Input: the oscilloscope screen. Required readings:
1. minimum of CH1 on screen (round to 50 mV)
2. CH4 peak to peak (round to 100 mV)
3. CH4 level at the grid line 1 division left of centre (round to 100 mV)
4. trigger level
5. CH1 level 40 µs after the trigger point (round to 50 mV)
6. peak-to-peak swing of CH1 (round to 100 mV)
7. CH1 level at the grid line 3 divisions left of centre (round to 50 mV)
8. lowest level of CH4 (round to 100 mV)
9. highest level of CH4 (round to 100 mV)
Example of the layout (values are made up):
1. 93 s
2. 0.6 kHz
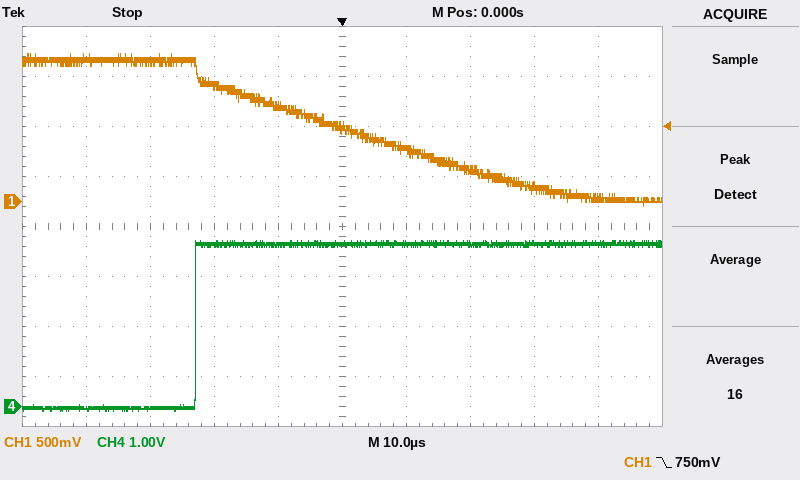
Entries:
1. -50 mV
2. 3.4 V
3. 3.2 V
4. 750 mV
5. 50 mV
6. 1.50 V
7. 1.40 V
8. -100 mV
9. 3.3 V
